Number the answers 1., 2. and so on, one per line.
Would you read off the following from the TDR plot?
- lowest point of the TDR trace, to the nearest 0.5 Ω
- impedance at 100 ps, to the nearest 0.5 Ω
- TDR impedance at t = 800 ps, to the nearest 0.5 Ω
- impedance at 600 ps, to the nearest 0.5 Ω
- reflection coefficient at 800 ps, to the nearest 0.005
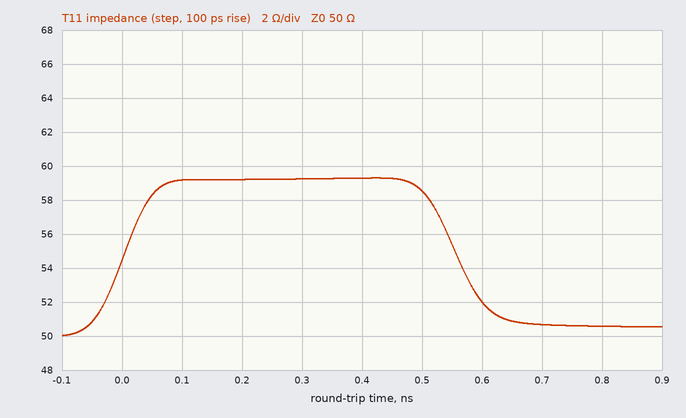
1. 50.0 Ω
2. 59.0 Ω
3. 50.5 Ω
4. 52.0 Ω
5. +0.005
